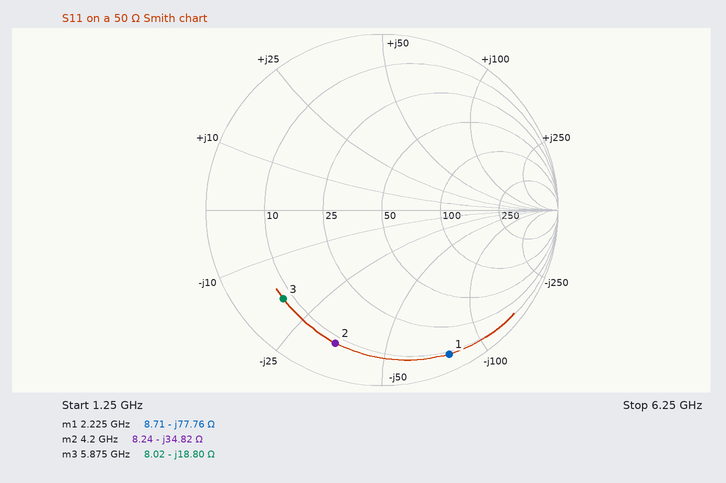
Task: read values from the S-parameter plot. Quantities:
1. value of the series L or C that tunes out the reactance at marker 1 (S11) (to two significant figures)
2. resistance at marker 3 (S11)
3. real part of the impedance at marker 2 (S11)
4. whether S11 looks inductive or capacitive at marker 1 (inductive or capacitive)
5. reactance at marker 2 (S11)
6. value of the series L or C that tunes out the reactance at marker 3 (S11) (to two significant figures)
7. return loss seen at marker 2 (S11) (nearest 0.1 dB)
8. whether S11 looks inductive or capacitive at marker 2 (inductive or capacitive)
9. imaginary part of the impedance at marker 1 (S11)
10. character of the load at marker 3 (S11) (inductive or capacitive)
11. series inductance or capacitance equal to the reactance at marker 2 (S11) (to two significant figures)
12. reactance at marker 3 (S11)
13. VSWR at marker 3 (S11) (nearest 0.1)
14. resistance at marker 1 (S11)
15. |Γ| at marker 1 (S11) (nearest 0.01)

5.6 nH
8.02 Ω
8.24 Ω
capacitive
-34.82 Ω
510 pH
1.9 dB
capacitive
-77.76 Ω
capacitive
1.1 pF
-18.80 Ω
7.1
8.71 Ω
0.90
